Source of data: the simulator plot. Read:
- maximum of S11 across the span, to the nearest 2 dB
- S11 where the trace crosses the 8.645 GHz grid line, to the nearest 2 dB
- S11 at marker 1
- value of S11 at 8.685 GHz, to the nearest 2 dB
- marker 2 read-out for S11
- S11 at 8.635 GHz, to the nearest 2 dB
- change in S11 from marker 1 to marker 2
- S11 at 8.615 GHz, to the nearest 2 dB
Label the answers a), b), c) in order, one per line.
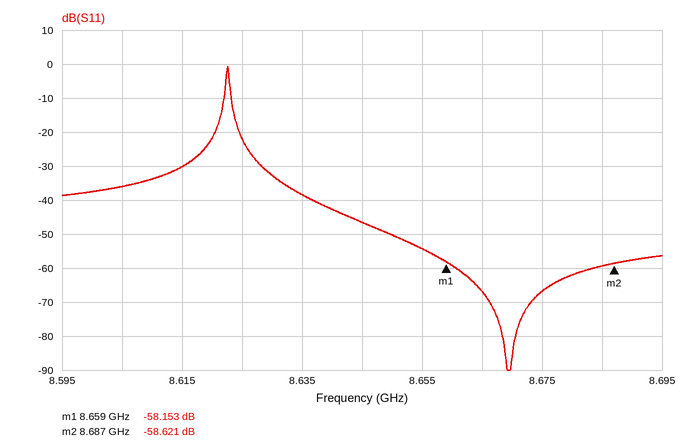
a) 0 dB
b) -46 dB
c) -58.153 dB
d) -60 dB
e) -58.621 dB
f) -38 dB
g) -0.468 dB
h) -30 dB
